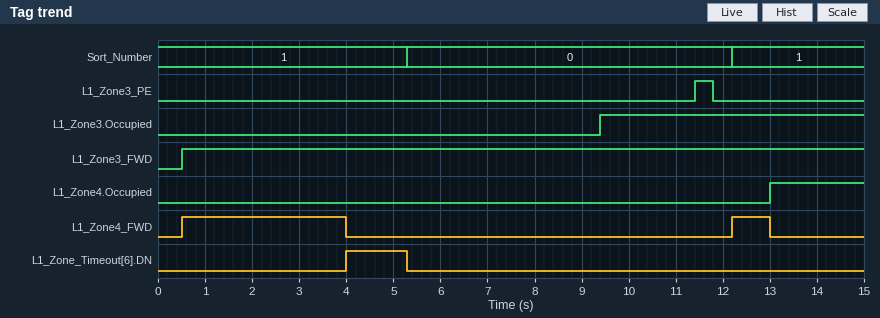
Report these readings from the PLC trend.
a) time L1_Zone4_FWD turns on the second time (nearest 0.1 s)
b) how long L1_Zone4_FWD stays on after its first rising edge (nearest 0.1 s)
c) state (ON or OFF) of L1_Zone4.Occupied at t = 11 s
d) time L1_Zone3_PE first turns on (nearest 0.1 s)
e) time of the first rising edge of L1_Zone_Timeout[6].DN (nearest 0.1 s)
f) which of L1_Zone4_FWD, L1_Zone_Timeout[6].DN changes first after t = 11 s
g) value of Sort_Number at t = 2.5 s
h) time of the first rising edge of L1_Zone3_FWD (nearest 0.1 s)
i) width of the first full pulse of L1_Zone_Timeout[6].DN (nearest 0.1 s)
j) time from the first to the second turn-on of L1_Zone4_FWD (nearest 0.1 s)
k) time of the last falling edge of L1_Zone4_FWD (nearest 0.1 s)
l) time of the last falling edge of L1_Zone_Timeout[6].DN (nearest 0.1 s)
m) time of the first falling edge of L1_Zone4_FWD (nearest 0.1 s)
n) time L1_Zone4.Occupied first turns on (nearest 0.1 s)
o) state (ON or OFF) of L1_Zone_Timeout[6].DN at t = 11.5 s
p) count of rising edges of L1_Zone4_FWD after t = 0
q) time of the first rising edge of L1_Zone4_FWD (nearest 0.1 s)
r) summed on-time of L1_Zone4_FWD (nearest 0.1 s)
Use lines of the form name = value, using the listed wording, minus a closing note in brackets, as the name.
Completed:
time L1_Zone4_FWD turns on the second time = 12.2 s
how long L1_Zone4_FWD stays on after its first rising edge = 3.5 s
state (ON or OFF) of L1_Zone4.Occupied at t = 11 s = OFF
time L1_Zone3_PE first turns on = 11.4 s
time of the first rising edge of L1_Zone_Timeout[6].DN = 4.0 s
which of L1_Zone4_FWD, L1_Zone_Timeout[6].DN changes first after t = 11 s = L1_Zone4_FWD
value of Sort_Number at t = 2.5 s = 1
time of the first rising edge of L1_Zone3_FWD = 0.5 s
width of the first full pulse of L1_Zone_Timeout[6].DN = 1.3 s
time from the first to the second turn-on of L1_Zone4_FWD = 11.7 s
time of the last falling edge of L1_Zone4_FWD = 13.0 s
time of the last falling edge of L1_Zone_Timeout[6].DN = 5.3 s
time of the first falling edge of L1_Zone4_FWD = 4.0 s
time L1_Zone4.Occupied first turns on = 13.0 s
state (ON or OFF) of L1_Zone_Timeout[6].DN at t = 11.5 s = OFF
count of rising edges of L1_Zone4_FWD after t = 0 = 2
time of the first rising edge of L1_Zone4_FWD = 0.5 s
summed on-time of L1_Zone4_FWD = 4.3 s
